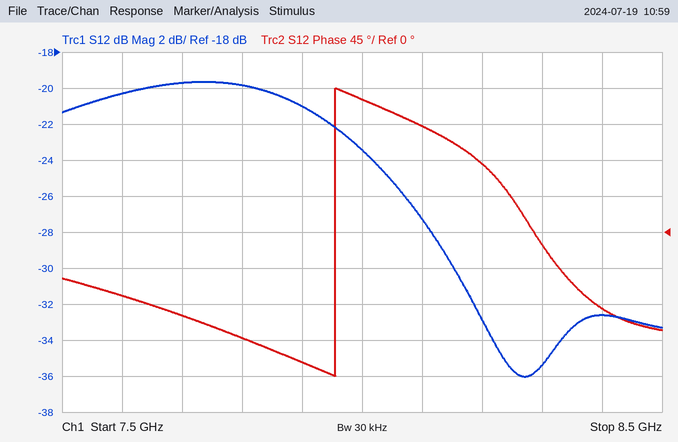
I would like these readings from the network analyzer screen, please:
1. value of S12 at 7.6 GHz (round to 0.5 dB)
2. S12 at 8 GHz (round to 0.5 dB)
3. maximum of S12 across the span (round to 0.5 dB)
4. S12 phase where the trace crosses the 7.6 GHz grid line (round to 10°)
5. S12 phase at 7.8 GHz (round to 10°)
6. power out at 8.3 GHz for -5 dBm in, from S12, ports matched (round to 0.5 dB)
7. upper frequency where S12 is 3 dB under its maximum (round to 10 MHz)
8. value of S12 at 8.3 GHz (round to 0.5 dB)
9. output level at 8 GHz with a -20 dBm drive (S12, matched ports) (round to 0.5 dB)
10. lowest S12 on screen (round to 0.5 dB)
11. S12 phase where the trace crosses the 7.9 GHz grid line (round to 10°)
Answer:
-20.5 dB
-23.5 dB
-19.5 dB
-80°
-130°
-40.5 dBm
7.97 GHz
-35.5 dB
-43.5 dBm
-36.0 dB
-160°
